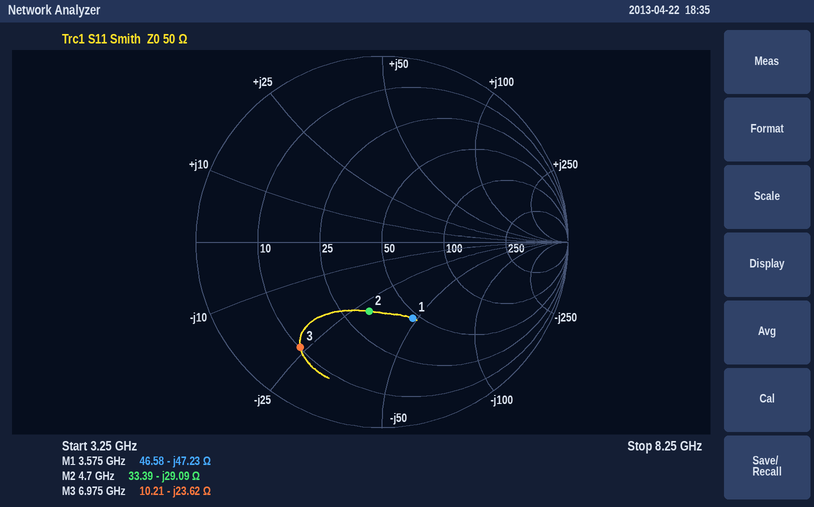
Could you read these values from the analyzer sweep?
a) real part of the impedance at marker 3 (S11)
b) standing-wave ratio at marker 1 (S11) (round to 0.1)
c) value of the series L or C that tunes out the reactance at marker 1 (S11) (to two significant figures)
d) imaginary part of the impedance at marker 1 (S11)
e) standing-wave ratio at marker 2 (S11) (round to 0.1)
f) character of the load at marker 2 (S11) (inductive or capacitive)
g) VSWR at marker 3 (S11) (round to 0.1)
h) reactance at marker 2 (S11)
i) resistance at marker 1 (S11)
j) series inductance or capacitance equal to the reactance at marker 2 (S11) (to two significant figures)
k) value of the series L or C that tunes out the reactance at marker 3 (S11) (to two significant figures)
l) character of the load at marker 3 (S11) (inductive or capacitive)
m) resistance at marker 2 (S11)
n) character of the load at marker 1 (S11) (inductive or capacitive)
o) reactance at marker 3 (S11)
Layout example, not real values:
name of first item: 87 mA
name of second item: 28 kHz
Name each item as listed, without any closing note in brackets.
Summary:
real part of the impedance at marker 3: 10.21 Ω
standing-wave ratio at marker 1 (S11): 2.6
value of the series L or C that tunes out the reactance at marker 1 (S11): 2.1 nH
imaginary part of the impedance at marker 1: -47.23 Ω
standing-wave ratio at marker 2 (S11): 2.2
character of the load at marker 2 (S11): capacitive
VSWR at marker 3 (S11): 6.0
reactance at marker 2: -29.09 Ω
resistance at marker 1: 46.58 Ω
series inductance or capacitance equal to the reactance at marker 2 (S11): 1.2 pF
value of the series L or C that tunes out the reactance at marker 3 (S11): 540 pH
character of the load at marker 3 (S11): capacitive
resistance at marker 2: 33.39 Ω
character of the load at marker 1 (S11): capacitive
reactance at marker 3: -23.62 Ω
